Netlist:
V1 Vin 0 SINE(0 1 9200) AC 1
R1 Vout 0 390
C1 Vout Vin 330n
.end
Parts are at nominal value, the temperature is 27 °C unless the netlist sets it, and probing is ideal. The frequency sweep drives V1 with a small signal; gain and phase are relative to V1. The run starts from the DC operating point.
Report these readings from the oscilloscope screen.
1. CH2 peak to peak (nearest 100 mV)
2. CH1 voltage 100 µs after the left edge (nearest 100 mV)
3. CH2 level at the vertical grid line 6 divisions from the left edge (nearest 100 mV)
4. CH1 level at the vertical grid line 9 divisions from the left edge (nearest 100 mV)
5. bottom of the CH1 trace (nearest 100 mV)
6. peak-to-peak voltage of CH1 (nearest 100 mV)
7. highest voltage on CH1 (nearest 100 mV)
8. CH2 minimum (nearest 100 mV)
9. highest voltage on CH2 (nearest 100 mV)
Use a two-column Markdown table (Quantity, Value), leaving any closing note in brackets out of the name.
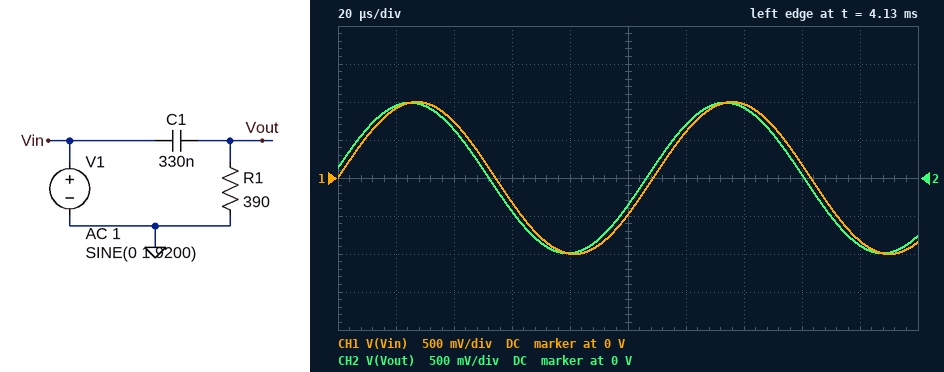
| Quantity | Value |
|---|---|
| CH2 peak to peak | 2.0 V |
| CH1 voltage 100 µs after the left edge | -500 mV |
| CH2 level at the vertical grid line 6 divisions from the left edge | 700 mV |
| CH1 level at the vertical grid line 9 divisions from the left edge | -800 mV |
| bottom of the CH1 trace | -1.0 V |
| peak-to-peak voltage of CH1 | 2.0 V |
| highest voltage on CH1 | 1.0 V |
| CH2 minimum | -1.0 V |
| highest voltage on CH2 | 1.0 V |
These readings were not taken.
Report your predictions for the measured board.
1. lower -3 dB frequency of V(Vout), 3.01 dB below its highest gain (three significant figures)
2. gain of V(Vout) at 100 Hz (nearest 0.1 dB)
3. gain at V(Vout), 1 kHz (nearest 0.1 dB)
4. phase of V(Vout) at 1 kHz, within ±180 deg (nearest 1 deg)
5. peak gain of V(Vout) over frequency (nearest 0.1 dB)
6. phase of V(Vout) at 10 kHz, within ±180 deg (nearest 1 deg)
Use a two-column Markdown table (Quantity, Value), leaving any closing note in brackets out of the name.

| Quantity | Value |
|---|---|
| lower -3 dB frequency of V(Vout), 3.01 dB below its highest gain | 1.24 kHz |
| gain of V(Vout) at 100 Hz | -21.9 dB |
| gain at V(Vout), 1 kHz | -4.0 dB |
| phase of V(Vout) at 1 kHz, within ±180 deg | 51 deg |
| peak gain of V(Vout) over frequency | 0 dB |
| phase of V(Vout) at 10 kHz, within ±180 deg | 7 deg |
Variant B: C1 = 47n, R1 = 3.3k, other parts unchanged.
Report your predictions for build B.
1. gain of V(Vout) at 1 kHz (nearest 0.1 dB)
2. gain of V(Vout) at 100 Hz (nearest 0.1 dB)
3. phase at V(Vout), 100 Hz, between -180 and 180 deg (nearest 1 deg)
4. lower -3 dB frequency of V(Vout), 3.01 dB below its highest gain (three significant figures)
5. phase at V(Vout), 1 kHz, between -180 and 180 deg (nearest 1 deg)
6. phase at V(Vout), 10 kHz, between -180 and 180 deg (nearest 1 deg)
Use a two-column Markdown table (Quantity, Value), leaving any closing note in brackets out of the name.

| Quantity | Value |
|---|---|
| gain of V(Vout) at 1 kHz | -3.1 dB |
| gain of V(Vout) at 100 Hz | -20.3 dB |
| phase at V(Vout), 100 Hz, between -180 and 180 deg | 84 deg |
| lower -3 dB frequency of V(Vout), 3.01 dB below its highest gain | 1.03 kHz |
| phase at V(Vout), 1 kHz, between -180 and 180 deg | 46 deg |
| phase at V(Vout), 10 kHz, between -180 and 180 deg | 6 deg |
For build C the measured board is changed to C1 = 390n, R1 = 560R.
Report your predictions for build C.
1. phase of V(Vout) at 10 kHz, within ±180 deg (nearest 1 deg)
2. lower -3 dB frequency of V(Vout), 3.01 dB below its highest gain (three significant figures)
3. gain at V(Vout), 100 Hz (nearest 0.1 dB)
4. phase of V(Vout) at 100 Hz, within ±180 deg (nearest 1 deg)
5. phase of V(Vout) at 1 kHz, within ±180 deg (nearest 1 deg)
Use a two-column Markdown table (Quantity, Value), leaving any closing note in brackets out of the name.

| Quantity | Value |
|---|---|
| phase of V(Vout) at 10 kHz, within ±180 deg | 4 deg |
| lower -3 dB frequency of V(Vout), 3.01 dB below its highest gain | 729 Hz |
| gain at V(Vout), 100 Hz | -17.3 dB |
| phase of V(Vout) at 100 Hz, within ±180 deg | 82 deg |
| phase of V(Vout) at 1 kHz, within ±180 deg | 36 deg |
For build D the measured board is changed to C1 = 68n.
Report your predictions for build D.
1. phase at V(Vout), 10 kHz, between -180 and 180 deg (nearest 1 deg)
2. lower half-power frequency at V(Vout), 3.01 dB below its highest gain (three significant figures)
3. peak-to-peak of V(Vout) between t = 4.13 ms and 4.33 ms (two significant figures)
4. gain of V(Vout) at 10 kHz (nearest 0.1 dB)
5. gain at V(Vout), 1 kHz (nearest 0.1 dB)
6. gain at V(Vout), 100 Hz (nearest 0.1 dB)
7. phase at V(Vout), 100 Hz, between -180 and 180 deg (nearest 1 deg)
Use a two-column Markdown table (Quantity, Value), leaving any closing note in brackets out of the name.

| Quantity | Value |
|---|---|
| phase at V(Vout), 10 kHz, between -180 and 180 deg | 31 deg |
| lower half-power frequency at V(Vout), 3.01 dB below its highest gain | 6.00 kHz |
| peak-to-peak of V(Vout) between t = 4.13 ms and 4.33 ms | 1.7 V |
| gain of V(Vout) at 10 kHz | -1.3 dB |
| gain at V(Vout), 1 kHz | -15.7 dB |
| gain at V(Vout), 100 Hz | -35.6 dB |
| phase at V(Vout), 100 Hz, between -180 and 180 deg | 89 deg |
